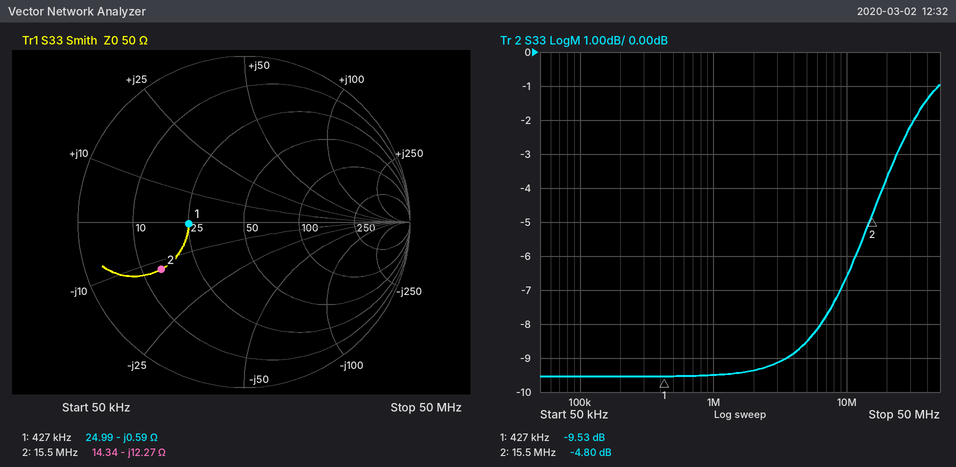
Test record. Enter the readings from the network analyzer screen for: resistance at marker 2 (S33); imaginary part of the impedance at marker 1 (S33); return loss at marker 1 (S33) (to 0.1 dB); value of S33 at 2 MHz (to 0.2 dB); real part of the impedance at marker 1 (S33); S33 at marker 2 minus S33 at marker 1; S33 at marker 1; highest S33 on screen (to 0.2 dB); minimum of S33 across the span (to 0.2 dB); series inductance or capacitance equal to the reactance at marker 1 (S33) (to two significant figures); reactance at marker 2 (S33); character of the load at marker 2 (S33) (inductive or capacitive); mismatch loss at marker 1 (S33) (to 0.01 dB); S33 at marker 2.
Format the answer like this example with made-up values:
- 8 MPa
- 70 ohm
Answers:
- 14.34 Ω
- -0.59 Ω
- 9.5 dB
- -9.4 dB
- 24.99 Ω
- 4.73 dB
- -9.53 dB
- -1.0 dB
- -9.6 dB
- 630 nF
- -12.27 Ω
- capacitive
- 0.51 dB
- -4.80 dB
